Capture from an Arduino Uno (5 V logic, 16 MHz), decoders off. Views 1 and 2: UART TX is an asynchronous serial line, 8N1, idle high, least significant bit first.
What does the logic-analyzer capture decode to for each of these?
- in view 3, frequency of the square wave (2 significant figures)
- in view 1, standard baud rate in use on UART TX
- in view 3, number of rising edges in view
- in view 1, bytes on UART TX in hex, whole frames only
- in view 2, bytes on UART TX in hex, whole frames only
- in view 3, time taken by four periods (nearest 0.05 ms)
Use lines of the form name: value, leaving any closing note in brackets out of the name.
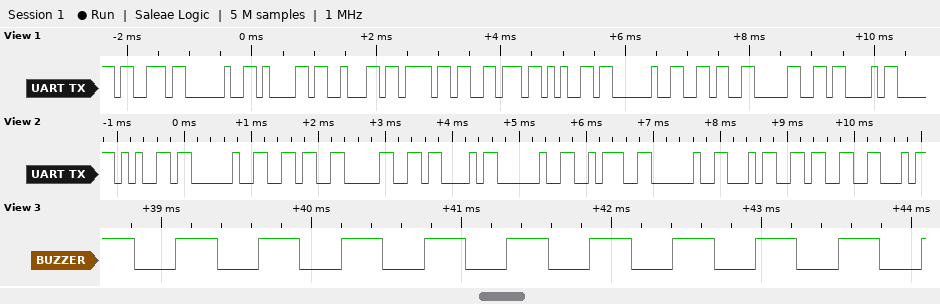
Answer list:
in view 3, frequency of the square wave: 1.8 kHz
in view 1, standard baud rate in use on UART TX: 9600 baud
in view 3, number of rising edges in view: 10
in view 1, bytes on UART TX in hex, whole frames only: 73 20 61 62 6F 76 65 20 36 30 43
in view 2, bytes on UART TX in hex, whole frames only: 65 20 36 30 43 20 3A 20 34 33
in view 3, time taken by four periods: 2.20 ms
